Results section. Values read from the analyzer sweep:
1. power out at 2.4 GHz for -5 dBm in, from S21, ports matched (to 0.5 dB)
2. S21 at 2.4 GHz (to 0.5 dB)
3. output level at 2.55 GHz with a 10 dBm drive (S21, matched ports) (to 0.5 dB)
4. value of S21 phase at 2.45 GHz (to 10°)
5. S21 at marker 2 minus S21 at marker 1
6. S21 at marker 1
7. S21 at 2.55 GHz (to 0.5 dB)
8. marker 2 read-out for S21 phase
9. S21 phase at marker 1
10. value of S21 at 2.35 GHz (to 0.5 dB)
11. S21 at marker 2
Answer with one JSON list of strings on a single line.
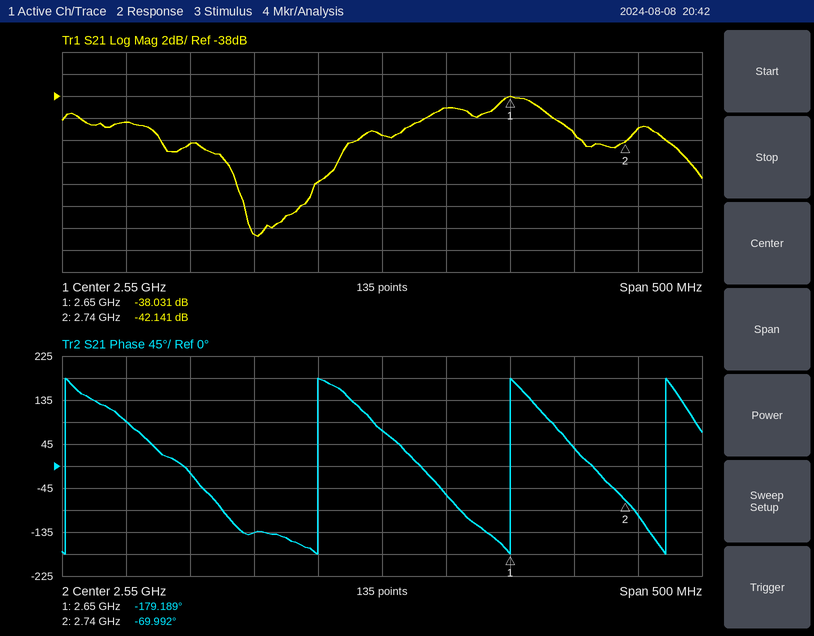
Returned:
["-47.5 dBm", "-42.5 dB", "-31.5 dBm", "-140°", "-4.110 dB", "-38.031 dB", "-41.5 dB", "-69.992°", "-179.189°", "-40.5 dB", "-42.141 dB"]
